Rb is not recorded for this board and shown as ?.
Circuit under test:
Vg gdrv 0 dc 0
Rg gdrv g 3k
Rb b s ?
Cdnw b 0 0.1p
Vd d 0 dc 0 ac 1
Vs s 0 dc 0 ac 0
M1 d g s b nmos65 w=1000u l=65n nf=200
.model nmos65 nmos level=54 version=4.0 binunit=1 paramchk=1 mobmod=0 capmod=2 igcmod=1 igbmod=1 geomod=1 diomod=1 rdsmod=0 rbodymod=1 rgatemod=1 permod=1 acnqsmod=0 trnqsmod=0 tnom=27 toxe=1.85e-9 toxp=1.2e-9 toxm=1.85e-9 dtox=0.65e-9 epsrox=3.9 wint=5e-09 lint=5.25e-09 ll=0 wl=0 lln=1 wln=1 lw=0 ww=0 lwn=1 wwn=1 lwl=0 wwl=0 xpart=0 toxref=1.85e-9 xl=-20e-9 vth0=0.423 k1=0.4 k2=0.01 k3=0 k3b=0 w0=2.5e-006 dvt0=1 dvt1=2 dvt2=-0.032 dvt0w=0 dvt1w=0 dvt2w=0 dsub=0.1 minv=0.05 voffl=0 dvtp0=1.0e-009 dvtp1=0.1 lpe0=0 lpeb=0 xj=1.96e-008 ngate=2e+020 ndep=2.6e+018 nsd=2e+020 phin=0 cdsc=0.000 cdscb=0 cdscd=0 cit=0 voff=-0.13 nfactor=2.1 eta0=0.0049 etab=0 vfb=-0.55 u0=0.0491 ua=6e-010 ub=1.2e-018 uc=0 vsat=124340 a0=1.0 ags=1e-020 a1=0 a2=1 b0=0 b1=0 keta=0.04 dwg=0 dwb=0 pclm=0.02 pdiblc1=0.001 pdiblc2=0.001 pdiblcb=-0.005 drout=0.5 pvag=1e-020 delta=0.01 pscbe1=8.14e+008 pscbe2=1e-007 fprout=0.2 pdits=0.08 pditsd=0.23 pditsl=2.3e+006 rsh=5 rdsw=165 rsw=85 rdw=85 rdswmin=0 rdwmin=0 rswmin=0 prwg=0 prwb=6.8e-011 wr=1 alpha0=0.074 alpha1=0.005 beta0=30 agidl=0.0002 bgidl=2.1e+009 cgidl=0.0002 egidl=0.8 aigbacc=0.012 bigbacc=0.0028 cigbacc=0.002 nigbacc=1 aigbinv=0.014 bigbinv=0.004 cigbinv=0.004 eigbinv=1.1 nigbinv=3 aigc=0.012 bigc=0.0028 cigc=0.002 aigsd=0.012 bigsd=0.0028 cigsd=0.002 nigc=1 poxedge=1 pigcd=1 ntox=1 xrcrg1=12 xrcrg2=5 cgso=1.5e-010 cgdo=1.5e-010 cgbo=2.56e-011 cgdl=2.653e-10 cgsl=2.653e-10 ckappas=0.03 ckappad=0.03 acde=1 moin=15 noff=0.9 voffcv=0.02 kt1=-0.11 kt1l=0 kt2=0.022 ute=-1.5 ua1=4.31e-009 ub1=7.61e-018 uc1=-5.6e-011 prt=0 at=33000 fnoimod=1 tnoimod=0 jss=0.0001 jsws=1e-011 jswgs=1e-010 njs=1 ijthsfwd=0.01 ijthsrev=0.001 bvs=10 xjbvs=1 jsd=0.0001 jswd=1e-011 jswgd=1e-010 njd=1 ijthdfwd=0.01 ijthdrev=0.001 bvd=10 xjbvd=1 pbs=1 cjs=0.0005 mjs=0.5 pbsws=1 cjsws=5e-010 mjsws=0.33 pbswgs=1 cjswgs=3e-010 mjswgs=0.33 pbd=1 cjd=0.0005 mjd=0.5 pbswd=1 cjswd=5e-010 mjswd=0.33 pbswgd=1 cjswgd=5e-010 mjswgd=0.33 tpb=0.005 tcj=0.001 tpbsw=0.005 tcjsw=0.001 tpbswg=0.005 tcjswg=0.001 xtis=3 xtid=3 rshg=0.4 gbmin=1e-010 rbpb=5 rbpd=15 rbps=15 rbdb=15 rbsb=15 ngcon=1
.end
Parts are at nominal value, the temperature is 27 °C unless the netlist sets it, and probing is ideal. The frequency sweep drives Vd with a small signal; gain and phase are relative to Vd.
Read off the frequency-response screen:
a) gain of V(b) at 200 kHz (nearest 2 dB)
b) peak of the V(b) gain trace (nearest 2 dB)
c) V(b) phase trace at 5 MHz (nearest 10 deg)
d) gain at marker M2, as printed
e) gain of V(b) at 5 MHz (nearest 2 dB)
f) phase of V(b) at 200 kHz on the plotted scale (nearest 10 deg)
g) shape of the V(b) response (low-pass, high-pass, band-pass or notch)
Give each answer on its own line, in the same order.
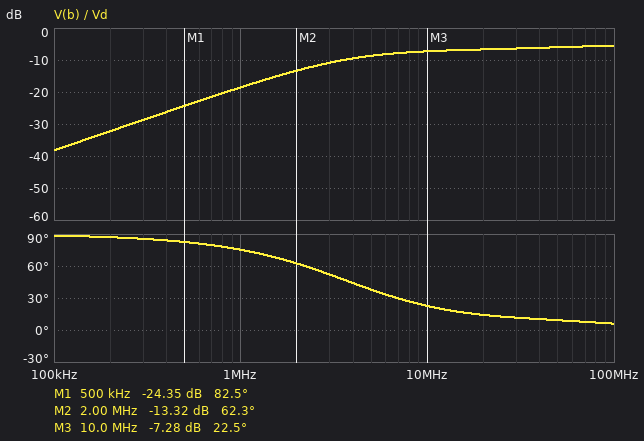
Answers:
-32 dB
-6 dB
40 deg
-13.32 dB
-8 dB
90 deg
high-pass
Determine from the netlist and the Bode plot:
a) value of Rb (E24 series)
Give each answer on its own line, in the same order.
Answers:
39 kΩ
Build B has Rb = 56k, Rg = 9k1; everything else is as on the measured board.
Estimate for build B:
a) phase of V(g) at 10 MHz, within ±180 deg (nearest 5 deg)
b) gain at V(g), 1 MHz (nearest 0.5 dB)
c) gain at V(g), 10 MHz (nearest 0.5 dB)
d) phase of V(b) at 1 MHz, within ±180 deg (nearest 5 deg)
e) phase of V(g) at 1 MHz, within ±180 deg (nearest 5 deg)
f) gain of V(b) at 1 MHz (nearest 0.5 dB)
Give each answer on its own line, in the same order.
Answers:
60 deg
-32.0 dB
-12.0 dB
70 deg
90 deg
-15.5 dB
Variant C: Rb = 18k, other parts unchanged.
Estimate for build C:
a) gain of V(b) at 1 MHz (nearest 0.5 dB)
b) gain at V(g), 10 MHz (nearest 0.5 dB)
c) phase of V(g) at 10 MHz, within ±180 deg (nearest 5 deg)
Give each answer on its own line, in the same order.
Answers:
-25.0 dB
-21.0 dB
85 deg
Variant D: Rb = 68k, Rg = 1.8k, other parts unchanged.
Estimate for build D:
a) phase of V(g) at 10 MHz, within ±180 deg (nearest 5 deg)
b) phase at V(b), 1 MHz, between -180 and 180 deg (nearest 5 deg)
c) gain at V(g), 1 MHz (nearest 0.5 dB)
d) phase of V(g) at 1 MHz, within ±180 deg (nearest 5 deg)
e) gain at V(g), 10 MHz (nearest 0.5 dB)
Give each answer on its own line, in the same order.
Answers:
85 deg
65 deg
-46.0 dB
95 deg
-24.5 dB
